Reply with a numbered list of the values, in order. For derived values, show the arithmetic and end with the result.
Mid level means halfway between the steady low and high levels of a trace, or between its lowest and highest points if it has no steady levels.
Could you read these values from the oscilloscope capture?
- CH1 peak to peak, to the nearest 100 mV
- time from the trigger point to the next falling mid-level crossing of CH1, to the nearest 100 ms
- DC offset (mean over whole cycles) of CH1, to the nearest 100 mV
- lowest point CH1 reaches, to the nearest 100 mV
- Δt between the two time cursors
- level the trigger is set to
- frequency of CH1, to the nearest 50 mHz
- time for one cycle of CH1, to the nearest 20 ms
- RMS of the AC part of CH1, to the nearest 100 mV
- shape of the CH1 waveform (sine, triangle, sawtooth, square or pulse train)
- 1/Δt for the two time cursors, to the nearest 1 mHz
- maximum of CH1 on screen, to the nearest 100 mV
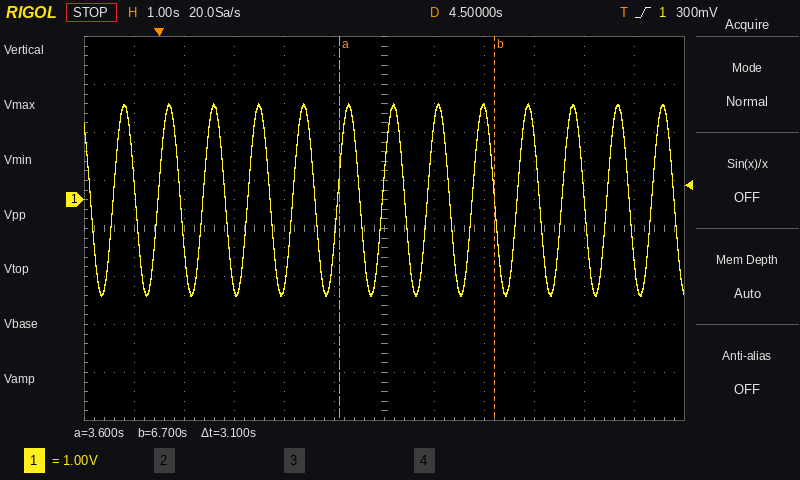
1. 2.0 V − (-2.0 V) = 4.0 V
2. 400 ms
3. (2.0 V + (-2.0 V)) / 2 ≈ 0.0 V
4. -2.0 V
5. 3.1 s
6. 300 mV
7. 1 / 900 ms ≈ 1.11 Hz, so 1.10 Hz to the nearest 50 mHz
8. 900 ms
9. 4.0 V / (2√2) ≈ 1.4 V
10. sine
11. 1 / 3.1 s ≈ 323 mHz
12. 2.0 V
